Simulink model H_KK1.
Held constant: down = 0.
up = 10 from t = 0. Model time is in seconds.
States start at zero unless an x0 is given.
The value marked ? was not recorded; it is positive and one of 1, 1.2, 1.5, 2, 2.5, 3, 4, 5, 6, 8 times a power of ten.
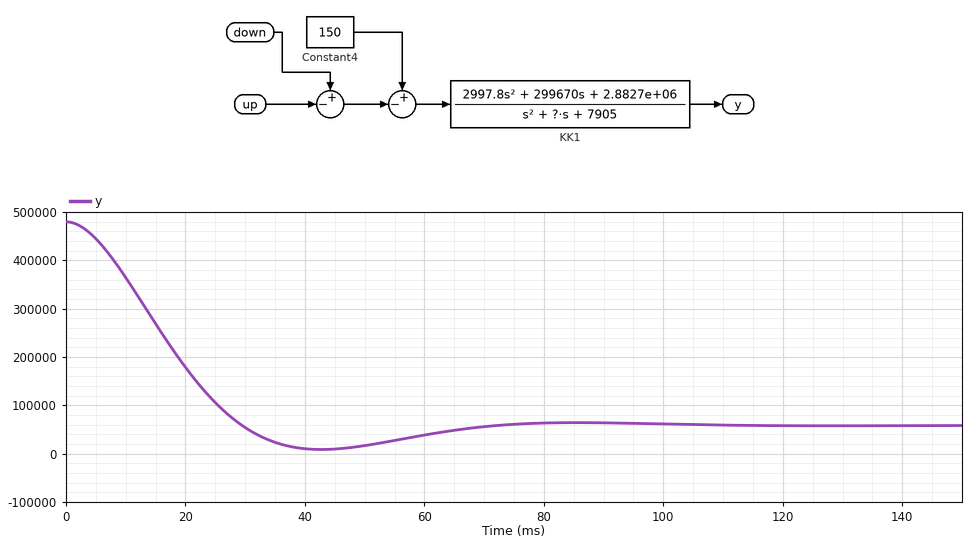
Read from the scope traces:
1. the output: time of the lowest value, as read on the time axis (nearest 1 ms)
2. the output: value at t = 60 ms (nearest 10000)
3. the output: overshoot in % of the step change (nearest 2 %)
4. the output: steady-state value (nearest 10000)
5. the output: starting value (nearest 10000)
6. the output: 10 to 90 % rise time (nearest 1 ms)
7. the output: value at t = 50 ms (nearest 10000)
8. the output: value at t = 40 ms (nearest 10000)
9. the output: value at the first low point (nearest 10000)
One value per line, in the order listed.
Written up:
43 ms
40000
12 %
60000
480000
20 ms
20000
10000
10000
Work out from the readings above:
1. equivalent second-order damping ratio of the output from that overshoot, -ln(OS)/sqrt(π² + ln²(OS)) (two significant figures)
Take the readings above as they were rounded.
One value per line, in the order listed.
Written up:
0.56
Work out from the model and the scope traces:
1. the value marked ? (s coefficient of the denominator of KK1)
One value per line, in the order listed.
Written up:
100
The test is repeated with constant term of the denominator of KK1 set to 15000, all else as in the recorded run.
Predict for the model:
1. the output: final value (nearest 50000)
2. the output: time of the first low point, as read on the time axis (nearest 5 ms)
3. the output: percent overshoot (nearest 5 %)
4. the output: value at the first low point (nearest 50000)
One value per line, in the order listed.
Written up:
50000
30 ms
25 %
-100000
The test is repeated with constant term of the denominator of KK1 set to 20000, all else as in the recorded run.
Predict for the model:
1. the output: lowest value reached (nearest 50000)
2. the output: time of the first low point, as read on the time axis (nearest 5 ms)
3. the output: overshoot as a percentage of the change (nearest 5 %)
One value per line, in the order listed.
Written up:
-100000
25 ms
30 %
